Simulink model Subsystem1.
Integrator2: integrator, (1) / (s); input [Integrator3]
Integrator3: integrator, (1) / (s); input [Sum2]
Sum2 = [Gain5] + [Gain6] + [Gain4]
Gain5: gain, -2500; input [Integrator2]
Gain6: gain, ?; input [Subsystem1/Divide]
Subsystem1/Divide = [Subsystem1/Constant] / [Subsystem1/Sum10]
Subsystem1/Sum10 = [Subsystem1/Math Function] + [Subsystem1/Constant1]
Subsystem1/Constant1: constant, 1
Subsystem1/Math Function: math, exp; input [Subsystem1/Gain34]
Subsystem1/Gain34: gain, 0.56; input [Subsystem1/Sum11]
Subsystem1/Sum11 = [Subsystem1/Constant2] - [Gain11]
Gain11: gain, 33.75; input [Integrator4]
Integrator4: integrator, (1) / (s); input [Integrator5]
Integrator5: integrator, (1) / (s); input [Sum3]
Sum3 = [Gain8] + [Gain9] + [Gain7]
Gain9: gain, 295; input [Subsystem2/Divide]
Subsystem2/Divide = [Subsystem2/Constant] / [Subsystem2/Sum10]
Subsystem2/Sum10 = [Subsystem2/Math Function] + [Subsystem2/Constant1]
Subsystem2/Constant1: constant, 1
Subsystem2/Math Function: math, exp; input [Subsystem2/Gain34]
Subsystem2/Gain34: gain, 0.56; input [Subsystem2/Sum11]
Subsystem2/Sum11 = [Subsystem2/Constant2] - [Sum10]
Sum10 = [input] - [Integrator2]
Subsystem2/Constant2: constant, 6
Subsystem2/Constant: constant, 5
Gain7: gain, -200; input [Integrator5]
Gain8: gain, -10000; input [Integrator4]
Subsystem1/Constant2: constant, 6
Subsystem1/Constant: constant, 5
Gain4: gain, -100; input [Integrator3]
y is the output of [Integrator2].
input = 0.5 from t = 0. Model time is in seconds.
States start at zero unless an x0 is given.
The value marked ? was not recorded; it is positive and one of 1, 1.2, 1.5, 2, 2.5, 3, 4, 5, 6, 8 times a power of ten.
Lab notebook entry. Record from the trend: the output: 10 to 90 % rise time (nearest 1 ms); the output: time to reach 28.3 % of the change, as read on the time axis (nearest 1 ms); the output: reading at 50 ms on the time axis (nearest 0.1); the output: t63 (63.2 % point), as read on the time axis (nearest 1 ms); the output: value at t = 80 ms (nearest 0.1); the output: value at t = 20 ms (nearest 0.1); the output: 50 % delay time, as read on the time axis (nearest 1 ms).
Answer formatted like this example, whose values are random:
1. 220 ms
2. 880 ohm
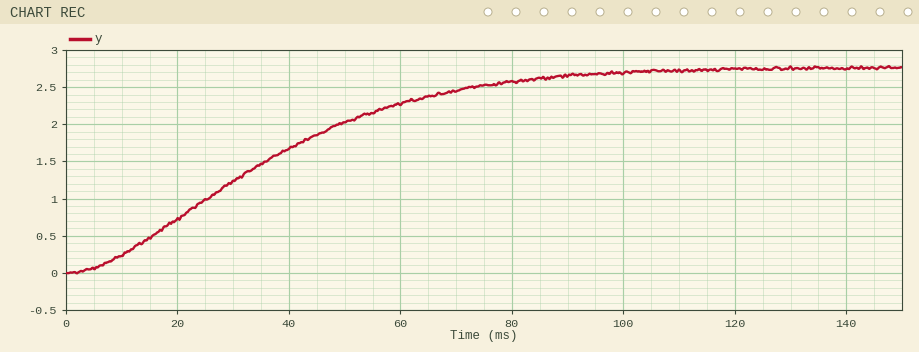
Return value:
1. 61 ms
2. 21 ms
3. 2.0
4. 42 ms
5. 2.6
6. 0.7
7. 33 ms
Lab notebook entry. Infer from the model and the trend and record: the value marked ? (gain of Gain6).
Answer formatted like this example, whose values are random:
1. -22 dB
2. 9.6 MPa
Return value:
1. 40000
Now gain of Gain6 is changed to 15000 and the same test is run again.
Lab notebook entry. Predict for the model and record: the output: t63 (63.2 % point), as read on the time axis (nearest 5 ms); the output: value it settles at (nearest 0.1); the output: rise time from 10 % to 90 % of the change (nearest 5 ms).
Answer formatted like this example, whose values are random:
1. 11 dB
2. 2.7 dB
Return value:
1. 45 ms
2. 1.1
3. 65 ms
